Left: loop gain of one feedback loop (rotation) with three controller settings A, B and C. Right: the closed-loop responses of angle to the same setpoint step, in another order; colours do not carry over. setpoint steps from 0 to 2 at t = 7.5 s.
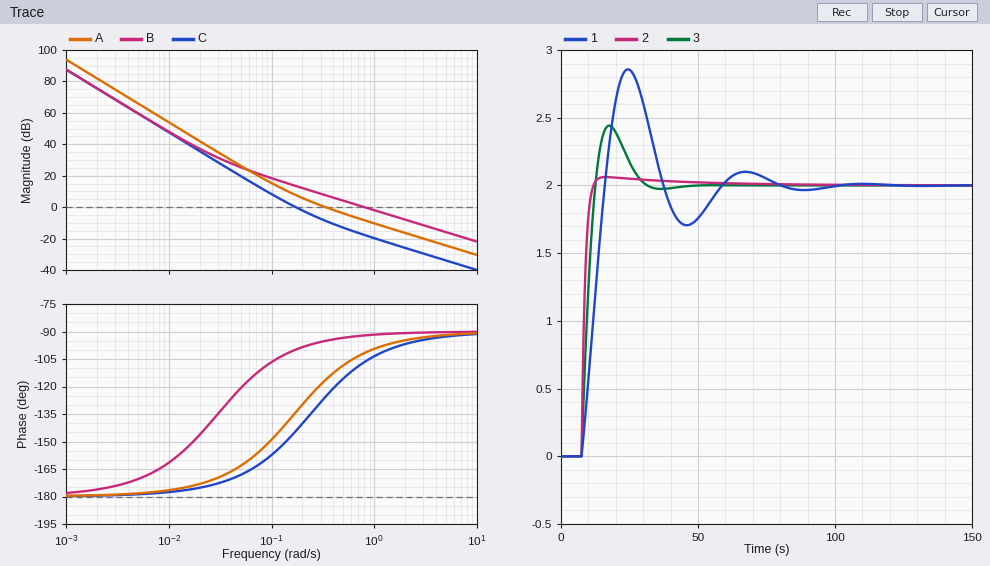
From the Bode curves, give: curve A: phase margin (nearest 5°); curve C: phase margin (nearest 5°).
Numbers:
65°
35°
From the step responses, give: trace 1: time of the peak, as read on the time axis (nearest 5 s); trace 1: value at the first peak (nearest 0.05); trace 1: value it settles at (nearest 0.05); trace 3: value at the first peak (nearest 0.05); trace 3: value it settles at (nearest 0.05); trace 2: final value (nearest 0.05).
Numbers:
25 s
2.85
2.00
2.45
2.00
2.00
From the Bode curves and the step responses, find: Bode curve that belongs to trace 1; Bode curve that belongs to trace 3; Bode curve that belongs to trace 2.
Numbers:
C
A
B
